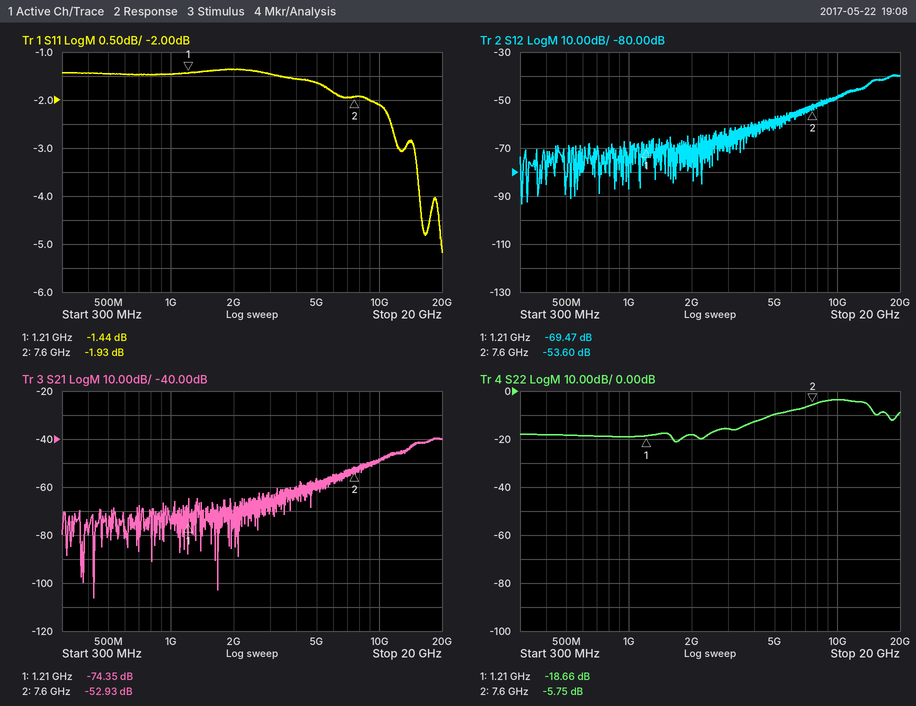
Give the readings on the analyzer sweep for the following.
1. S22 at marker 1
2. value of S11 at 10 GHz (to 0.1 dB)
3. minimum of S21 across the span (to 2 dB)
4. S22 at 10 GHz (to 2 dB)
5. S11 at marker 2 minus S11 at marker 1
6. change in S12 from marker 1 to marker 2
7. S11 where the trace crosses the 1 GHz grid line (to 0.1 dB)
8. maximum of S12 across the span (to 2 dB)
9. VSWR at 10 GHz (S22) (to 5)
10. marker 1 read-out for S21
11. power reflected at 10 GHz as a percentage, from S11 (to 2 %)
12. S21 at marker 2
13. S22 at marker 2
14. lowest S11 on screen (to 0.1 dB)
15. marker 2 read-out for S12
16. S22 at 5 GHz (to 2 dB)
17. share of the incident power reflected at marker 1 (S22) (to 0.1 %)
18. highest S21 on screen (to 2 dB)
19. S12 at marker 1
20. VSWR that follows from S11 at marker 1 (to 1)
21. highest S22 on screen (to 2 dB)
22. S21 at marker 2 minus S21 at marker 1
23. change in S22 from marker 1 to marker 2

-18.66 dB
-2.1 dB
-106 dB
-4 dB
-0.49 dB
15.87 dB
-1.5 dB
-40 dB
5
-74.35 dB
62 %
-52.93 dB
-5.75 dB
-5.2 dB
-53.60 dB
-10 dB
1.4 %
-40 dB
-69.47 dB
12
-4 dB
21.42 dB
12.91 dB
